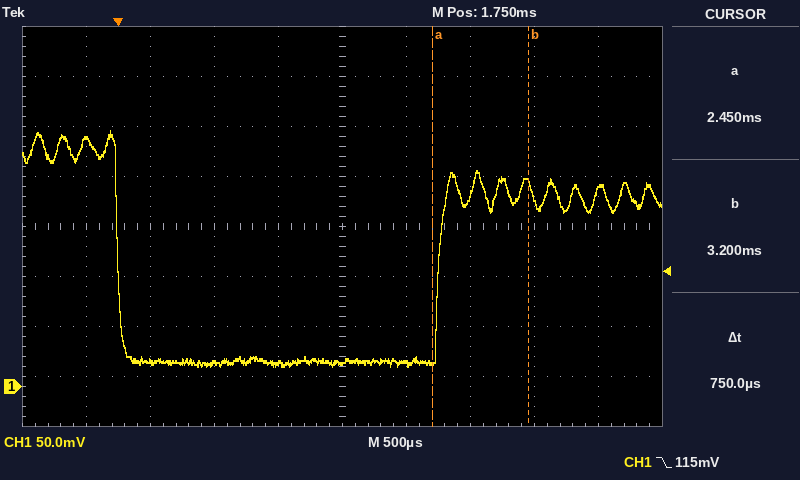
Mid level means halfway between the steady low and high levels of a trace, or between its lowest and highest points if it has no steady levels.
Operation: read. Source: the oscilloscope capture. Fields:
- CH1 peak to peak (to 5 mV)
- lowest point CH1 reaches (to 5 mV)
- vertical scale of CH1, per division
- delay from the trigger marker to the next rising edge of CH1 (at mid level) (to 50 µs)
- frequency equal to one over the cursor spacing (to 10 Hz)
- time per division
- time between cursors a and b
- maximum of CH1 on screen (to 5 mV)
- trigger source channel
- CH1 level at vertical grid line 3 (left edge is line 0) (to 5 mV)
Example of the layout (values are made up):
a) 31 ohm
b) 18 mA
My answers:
a) 235 mV
b) 20 mV
c) 50 mV
d) 2.50 ms
e) 1.33 kHz
f) 500 µs
g) 750 µs
h) 255 mV
i) CH1
j) 25 mV
